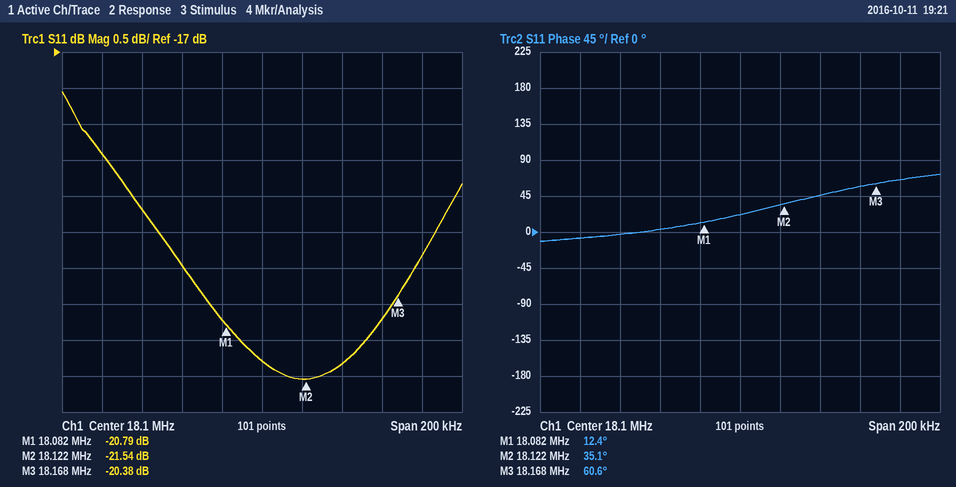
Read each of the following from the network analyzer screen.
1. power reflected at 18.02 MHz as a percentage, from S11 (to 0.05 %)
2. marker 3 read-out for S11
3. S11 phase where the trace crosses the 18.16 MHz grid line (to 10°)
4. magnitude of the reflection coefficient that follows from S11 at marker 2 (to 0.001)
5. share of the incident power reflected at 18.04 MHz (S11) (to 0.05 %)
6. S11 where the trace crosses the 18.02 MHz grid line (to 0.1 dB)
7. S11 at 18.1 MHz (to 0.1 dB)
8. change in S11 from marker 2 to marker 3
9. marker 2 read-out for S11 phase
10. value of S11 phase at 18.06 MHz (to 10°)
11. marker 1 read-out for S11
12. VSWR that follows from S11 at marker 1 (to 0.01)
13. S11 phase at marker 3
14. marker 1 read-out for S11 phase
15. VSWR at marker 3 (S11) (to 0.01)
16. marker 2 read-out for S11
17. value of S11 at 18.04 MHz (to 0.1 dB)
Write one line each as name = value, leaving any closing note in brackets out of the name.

power reflected at 18.02 MHz as a percentage, from S11 = 1.45 %
marker 3 read-out for S11 = -20.38 dB
S11 phase where the trace crosses the 18.16 MHz grid line = 60°
magnitude of the reflection coefficient that follows from S11 at marker 2 = 0.084
share of the incident power reflected at 18.04 MHz (S11) = 1.20 %
S11 where the trace crosses the 18.02 MHz grid line = -18.4 dB
S11 at 18.1 MHz = -21.3 dB
change in S11 from marker 2 to marker 3 = 1.16 dB
marker 2 read-out for S11 phase = 35.1°
value of S11 phase at 18.06 MHz = 0°
marker 1 read-out for S11 = -20.79 dB
VSWR that follows from S11 at marker 1 = 1.20
S11 phase at marker 3 = 60.6°
marker 1 read-out for S11 phase = 12.4°
VSWR at marker 3 (S11) = 1.21
marker 2 read-out for S11 = -21.54 dB
value of S11 at 18.04 MHz = -19.2 dB
